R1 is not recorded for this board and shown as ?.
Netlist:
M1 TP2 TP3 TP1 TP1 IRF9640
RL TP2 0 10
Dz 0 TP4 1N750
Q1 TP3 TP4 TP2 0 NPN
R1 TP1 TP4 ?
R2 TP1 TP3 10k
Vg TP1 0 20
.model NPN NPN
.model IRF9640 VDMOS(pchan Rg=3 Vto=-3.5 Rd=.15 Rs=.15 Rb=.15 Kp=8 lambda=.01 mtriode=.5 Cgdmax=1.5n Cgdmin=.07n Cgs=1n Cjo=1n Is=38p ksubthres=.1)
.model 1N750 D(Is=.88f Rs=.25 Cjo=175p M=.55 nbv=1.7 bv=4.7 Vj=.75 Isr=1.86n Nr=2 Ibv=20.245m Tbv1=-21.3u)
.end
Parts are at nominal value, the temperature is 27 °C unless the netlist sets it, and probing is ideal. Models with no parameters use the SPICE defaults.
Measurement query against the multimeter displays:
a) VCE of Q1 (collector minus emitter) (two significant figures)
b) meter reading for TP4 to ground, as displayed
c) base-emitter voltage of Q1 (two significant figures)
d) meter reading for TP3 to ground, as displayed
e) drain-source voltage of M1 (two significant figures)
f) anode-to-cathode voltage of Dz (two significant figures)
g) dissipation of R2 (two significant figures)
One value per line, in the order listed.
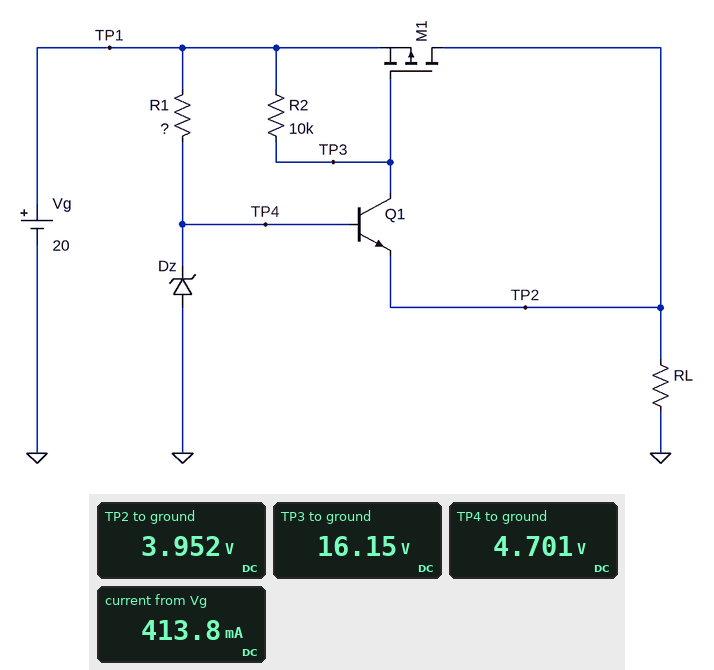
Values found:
12 V
4.701 V
750 mV
16.15 V
-16 V
-4.7 V
1.5 mW
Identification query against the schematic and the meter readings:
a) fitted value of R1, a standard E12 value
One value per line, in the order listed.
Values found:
820 Ω
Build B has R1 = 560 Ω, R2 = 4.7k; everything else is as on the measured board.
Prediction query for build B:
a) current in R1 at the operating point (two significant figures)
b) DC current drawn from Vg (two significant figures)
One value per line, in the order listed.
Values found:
27 mA
420 mA
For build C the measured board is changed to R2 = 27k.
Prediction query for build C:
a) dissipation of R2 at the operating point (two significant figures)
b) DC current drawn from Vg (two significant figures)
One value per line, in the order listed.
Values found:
550 µW
420 mA
